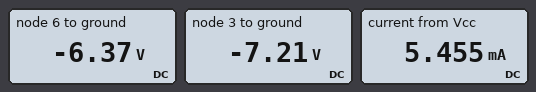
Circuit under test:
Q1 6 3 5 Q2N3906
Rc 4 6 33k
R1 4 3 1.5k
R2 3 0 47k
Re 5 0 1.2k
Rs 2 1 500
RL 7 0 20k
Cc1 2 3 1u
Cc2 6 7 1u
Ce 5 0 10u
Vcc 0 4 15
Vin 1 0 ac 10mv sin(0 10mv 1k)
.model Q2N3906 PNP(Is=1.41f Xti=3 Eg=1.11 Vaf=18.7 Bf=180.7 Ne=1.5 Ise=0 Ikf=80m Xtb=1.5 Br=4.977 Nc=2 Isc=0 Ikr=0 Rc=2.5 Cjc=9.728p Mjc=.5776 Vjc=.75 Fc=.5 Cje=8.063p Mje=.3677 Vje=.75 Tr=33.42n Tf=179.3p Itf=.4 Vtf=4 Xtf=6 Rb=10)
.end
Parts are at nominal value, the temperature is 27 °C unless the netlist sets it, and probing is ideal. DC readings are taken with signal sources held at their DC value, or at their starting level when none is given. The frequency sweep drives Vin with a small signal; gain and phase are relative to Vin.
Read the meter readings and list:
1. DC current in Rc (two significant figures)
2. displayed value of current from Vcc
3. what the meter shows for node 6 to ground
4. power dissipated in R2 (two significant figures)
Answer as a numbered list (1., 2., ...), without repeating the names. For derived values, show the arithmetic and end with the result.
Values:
1. (-6.37 V - (-15 V)) / 33 kΩ = 260 µA
2. 5.455 mA
3. -6.37 V
4. (0 V - (-7.21 V))^2 / 47 kΩ = 1.1 mW
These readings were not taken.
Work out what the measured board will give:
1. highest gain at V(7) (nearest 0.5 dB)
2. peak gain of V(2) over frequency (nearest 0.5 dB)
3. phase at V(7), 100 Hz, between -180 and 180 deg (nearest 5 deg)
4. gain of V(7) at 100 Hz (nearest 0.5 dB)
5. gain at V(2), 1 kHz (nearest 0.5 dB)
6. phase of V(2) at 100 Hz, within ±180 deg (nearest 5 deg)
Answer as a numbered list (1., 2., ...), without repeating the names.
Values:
1. -21.5 dB
2. 0 dB
3. 0 deg
4. -21.5 dB
5. -10.0 dB
6. -15 deg
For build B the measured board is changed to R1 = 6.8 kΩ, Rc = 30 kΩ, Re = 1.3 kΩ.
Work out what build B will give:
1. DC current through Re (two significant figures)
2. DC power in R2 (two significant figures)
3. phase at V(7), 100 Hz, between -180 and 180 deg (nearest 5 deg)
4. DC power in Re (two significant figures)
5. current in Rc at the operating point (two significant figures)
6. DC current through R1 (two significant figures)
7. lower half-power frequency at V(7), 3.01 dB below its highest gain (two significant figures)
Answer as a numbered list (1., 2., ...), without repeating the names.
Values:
1. 2.0 mA
2. 250 µW
3. -5 deg
4. 5.4 mW
5. 410 µA
6. 1.7 mA
7. 17 Hz
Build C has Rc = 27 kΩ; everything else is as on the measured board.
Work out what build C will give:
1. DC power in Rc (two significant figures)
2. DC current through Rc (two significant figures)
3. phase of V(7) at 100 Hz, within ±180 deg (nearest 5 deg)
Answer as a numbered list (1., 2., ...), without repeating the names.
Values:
1. 2.7 mW
2. 320 µA
3. 0 deg
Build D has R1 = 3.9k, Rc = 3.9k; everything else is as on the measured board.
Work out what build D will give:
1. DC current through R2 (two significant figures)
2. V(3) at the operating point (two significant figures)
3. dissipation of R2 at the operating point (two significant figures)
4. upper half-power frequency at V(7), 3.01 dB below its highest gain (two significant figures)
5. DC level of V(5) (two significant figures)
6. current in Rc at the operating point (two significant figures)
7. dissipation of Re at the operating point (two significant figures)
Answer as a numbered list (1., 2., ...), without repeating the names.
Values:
1. 130 µA
2. -6.3 V
3. 830 µW
4. 380 Hz
5. -5.5 V
6. 2.4 mA
7. 25 mW
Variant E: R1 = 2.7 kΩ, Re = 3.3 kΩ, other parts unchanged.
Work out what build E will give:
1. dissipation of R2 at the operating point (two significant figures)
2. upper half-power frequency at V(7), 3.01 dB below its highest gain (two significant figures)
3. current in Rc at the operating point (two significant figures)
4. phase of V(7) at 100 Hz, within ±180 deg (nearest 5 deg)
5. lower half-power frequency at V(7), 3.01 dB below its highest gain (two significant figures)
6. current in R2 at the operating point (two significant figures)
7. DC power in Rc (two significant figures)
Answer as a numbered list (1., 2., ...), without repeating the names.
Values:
1. 1.6 mW
2. 360 Hz
3. 220 µA
4. -5 deg
5. 14 Hz
6. 180 µA
7. 1.5 mW
